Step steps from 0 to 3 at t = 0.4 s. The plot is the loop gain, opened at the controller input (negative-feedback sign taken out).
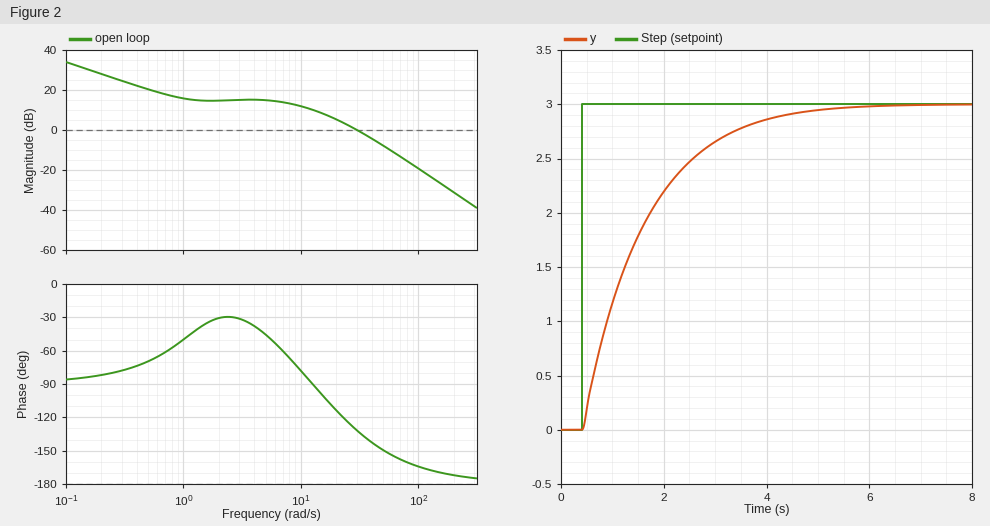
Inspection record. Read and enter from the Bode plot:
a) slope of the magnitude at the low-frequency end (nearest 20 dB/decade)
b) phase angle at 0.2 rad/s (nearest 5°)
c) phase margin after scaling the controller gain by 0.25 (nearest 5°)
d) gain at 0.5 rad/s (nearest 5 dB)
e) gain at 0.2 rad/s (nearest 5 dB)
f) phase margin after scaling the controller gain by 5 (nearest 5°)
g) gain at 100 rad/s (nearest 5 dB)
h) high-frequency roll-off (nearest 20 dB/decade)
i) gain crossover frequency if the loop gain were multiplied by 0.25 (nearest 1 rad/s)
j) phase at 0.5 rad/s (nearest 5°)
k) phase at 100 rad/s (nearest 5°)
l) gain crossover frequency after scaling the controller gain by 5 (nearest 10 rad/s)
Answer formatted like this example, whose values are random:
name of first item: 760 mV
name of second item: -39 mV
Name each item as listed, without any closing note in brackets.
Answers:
slope of the magnitude at the low-frequency end: -20 dB/decade
phase angle at 0.2 rad/s: -80°
phase margin after scaling the controller gain by 0.25: 105°
gain at 0.5 rad/s: 20 dB
gain at 0.2 rad/s: 30 dB
phase margin after scaling the controller gain by 5: 20°
gain at 100 rad/s: -20 dB
high-frequency roll-off: -40 dB/decade
gain crossover frequency if the loop gain were multiplied by 0.25: 10 rad/s
phase at 0.5 rad/s: -70°
phase at 100 rad/s: -165°
gain crossover frequency after scaling the controller gain by 5: 70 rad/s
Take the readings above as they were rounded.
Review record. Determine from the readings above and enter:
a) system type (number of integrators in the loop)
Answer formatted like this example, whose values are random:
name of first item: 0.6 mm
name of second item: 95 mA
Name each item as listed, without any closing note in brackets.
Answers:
system type: 1
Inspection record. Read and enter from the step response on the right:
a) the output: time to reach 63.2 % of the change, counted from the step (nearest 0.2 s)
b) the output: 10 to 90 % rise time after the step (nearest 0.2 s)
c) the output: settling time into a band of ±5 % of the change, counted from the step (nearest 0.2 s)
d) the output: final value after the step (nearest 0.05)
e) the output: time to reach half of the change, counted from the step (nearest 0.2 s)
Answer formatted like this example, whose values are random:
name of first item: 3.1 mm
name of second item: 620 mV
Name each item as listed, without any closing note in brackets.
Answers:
the output: time to reach 63.2 % of the change, counted from the step: 1.2 s
the output: 10 to 90 % rise time after the step: 2.6 s
the output: settling time into a band of ±5 % of the change, counted from the step: 3.6 s
the output: final value after the step: 3.00
the output: time to reach half of the change, counted from the step: 0.8 s
